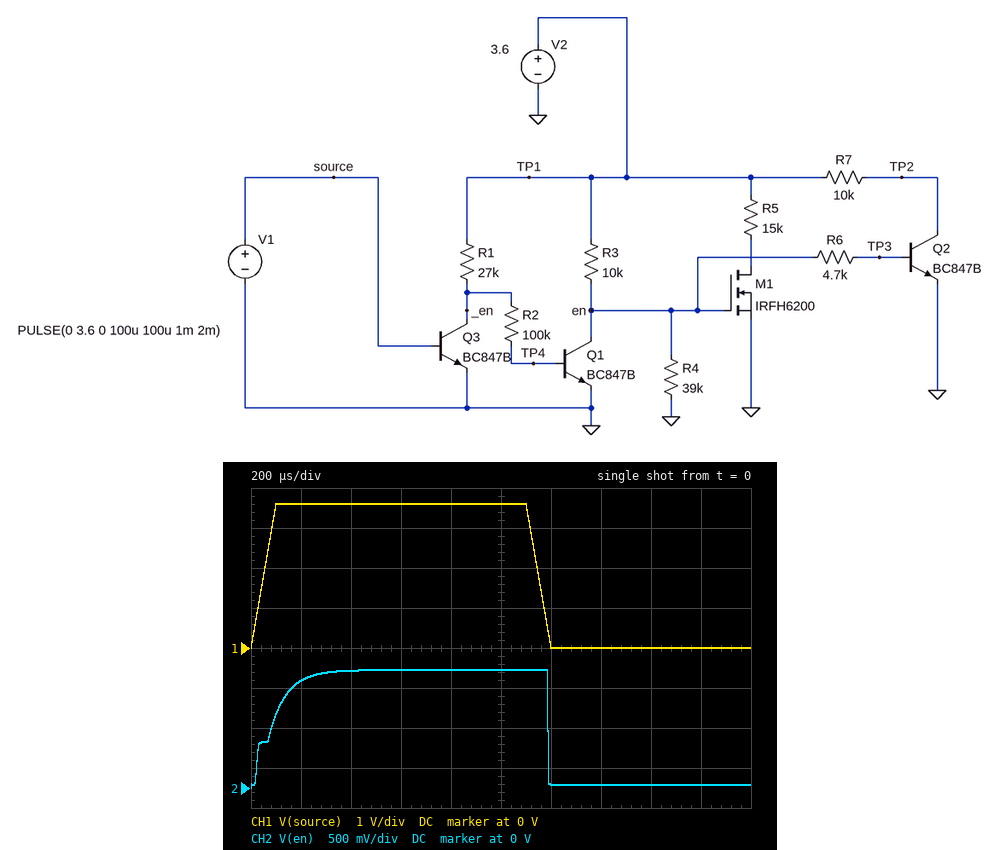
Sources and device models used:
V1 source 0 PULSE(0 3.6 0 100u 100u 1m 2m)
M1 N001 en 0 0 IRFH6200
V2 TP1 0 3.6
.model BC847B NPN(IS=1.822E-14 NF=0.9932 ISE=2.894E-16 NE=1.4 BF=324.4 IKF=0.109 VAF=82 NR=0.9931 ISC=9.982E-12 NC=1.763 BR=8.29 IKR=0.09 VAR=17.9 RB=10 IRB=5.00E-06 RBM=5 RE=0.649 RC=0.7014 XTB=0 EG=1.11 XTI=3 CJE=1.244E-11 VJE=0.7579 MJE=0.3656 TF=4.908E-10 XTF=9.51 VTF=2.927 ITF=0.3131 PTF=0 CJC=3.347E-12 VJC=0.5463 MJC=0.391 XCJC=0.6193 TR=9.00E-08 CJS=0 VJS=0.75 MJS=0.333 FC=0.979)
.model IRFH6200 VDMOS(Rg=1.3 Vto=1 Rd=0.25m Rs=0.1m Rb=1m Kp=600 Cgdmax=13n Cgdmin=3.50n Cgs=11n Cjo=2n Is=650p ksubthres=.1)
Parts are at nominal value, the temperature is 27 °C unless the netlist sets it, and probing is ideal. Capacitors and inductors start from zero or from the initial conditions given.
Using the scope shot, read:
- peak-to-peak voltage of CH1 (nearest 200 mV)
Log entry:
3.6 V
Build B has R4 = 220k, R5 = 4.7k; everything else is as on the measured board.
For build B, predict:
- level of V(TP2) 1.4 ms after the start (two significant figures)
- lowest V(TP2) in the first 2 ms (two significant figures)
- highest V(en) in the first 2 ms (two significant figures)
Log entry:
3.6 V
9.4 mV
1.6 V
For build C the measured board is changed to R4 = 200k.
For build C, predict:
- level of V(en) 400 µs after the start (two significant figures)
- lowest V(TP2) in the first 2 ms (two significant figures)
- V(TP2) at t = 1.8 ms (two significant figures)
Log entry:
1.6 V
9.4 mV
3.6 V
